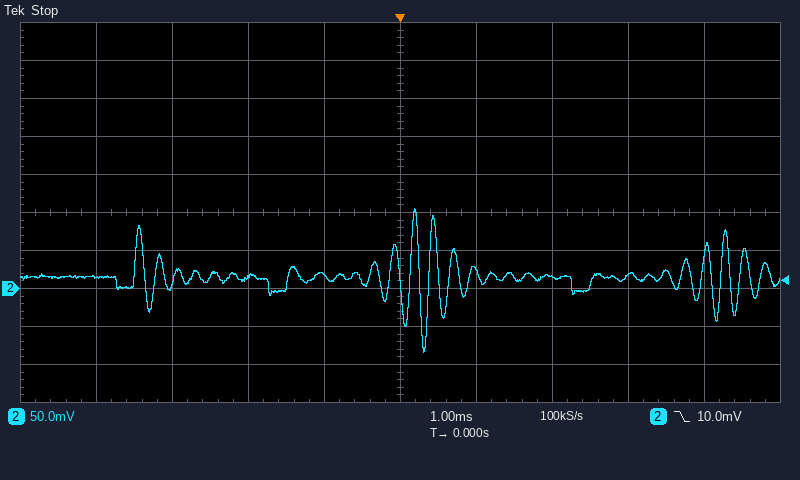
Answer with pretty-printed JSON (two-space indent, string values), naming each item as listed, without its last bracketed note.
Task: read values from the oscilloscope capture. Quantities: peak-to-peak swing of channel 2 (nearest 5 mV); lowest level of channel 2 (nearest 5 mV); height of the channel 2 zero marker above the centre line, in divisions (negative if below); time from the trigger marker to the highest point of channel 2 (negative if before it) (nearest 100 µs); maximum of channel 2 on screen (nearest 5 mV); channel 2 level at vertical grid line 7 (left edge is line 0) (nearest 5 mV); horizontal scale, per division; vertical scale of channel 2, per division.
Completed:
{
  "peak-to-peak swing of channel 2": "190 mV",
  "lowest level of channel 2": "-85 mV",
  "height of the channel 2 zero marker above the centre line, in divisions": "-2.0 div",
  "time from the trigger marker to the highest point of channel 2 (negative if before it)": "+200 µs",
  "maximum of channel 2 on screen": "105 mV",
  "channel 2 level at vertical grid line 7 (left edge is line 0)": "15 mV",
  "horizontal scale, per division": "1 ms",
  "vertical scale of channel 2, per division": "50 mV"
}
